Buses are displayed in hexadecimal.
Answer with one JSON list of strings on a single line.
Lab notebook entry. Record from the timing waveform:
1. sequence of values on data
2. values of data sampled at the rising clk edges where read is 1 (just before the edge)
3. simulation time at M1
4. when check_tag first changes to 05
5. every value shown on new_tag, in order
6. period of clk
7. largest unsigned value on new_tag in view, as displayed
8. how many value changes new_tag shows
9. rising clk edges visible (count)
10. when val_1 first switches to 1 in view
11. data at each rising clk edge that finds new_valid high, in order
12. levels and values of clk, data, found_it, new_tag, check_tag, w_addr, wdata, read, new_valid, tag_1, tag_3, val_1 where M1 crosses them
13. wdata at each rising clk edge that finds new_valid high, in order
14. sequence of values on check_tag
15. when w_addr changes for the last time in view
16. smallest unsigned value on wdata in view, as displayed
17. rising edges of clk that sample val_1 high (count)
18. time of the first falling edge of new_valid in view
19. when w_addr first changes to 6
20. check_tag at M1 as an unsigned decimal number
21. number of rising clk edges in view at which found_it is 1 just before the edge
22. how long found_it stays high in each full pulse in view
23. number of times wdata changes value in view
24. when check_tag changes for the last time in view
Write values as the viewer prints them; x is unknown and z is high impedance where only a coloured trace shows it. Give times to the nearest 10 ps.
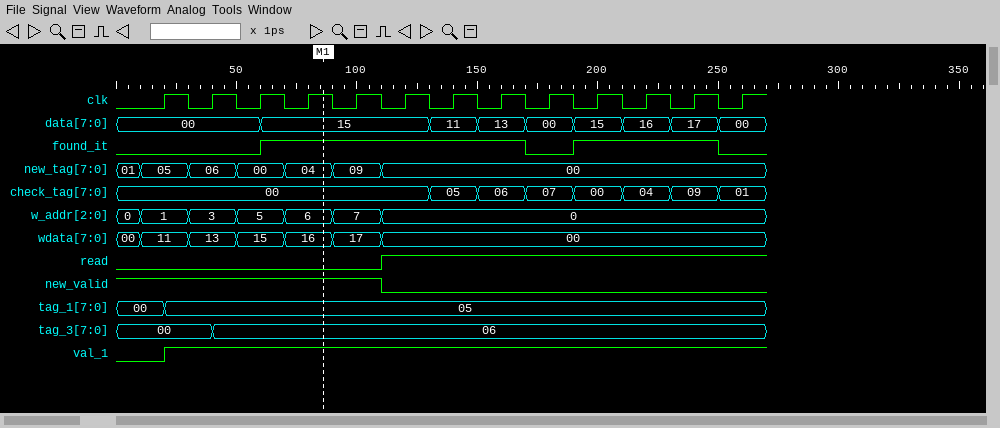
["00, 15, 11, 13, 00, 15, 16, 17, 00", "15, 11, 13, 00, 15, 16, 17, 00", "90 ps", "130 ps", "01, 05, 06, 00, 04, 09, 00", "20 ps", "09", "6", "13", "20 ps", "00, 00, 00, 15, 15", "clk=1, data=15, found_it=1, new_tag=04, check_tag=00, w_addr=6, wdata=16, read=0, new_valid=1, tag_1=05, tag_3=06, val_1=1", "11, 13, 15, 16, 17", "00, 05, 06, 07, 00, 04, 09, 01", "110 ps", "00", "12", "110 ps", "70 ps", "0", "8", "110 ps, 60 ps", "6", "250 ps"]
